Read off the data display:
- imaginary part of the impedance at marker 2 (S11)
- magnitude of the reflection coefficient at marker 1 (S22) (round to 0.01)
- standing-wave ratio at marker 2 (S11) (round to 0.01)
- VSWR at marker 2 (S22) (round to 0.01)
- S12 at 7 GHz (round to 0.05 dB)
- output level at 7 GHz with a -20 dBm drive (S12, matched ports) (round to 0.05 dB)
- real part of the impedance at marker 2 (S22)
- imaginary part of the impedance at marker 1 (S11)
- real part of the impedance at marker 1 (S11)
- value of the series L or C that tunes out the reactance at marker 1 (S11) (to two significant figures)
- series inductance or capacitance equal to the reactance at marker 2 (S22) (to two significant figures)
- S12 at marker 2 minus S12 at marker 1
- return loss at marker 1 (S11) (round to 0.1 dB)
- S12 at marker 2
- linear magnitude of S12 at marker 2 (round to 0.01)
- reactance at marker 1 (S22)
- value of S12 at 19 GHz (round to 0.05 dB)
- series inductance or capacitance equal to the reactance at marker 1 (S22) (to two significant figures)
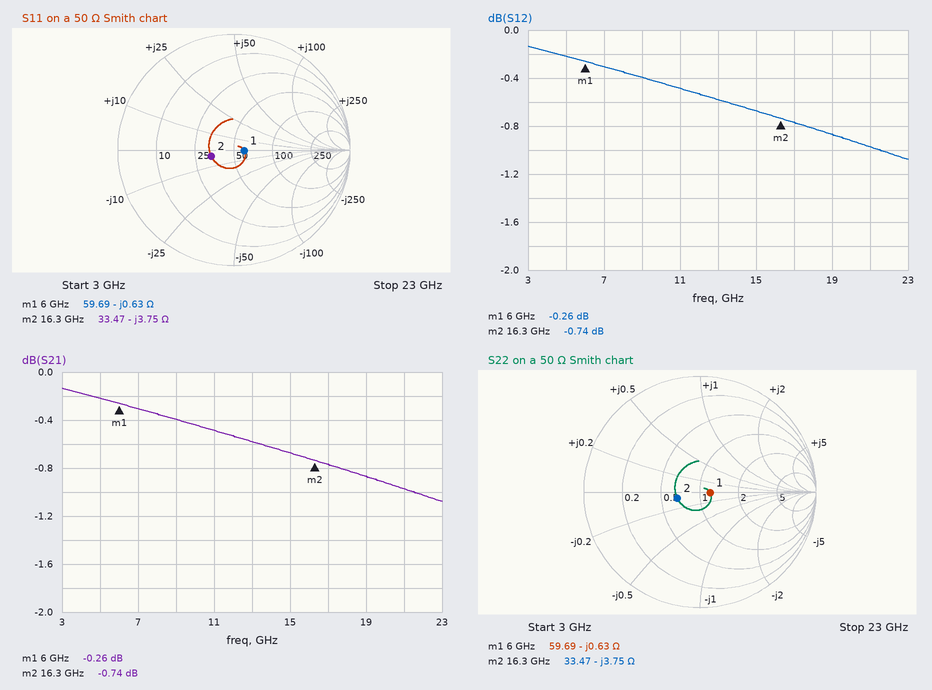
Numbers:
-3.75 Ω
0.09
1.51
1.51
-0.30 dB
-20.30 dBm
33.47 Ω
-0.63 Ω
59.69 Ω
17 pH
2.6 pF
-0.48 dB
21.1 dB
-0.74 dB
0.92
-0.63 Ω
-0.85 dB
42 pF
